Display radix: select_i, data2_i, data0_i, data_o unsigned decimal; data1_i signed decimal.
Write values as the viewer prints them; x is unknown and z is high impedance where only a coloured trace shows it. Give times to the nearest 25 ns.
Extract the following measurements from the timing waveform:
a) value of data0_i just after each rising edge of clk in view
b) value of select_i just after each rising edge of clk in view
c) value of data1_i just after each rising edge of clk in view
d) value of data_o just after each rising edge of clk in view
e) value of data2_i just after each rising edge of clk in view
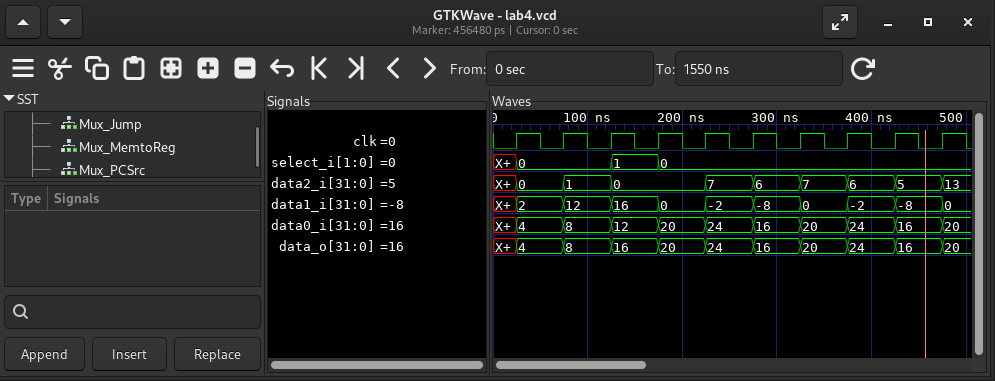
4, 8, 12, 20, 24, 16, 20, 24, 16, 20
0, 0, 1, 0, 0, 0, 0, 0, 0, 0
2, 12, 16, 0, -2, -8, 0, -2, -8, 0
4, 8, 16, 20, 24, 16, 20, 24, 16, 20
0, 1, 0, 0, 7, 6, 7, 6, 5, 13
